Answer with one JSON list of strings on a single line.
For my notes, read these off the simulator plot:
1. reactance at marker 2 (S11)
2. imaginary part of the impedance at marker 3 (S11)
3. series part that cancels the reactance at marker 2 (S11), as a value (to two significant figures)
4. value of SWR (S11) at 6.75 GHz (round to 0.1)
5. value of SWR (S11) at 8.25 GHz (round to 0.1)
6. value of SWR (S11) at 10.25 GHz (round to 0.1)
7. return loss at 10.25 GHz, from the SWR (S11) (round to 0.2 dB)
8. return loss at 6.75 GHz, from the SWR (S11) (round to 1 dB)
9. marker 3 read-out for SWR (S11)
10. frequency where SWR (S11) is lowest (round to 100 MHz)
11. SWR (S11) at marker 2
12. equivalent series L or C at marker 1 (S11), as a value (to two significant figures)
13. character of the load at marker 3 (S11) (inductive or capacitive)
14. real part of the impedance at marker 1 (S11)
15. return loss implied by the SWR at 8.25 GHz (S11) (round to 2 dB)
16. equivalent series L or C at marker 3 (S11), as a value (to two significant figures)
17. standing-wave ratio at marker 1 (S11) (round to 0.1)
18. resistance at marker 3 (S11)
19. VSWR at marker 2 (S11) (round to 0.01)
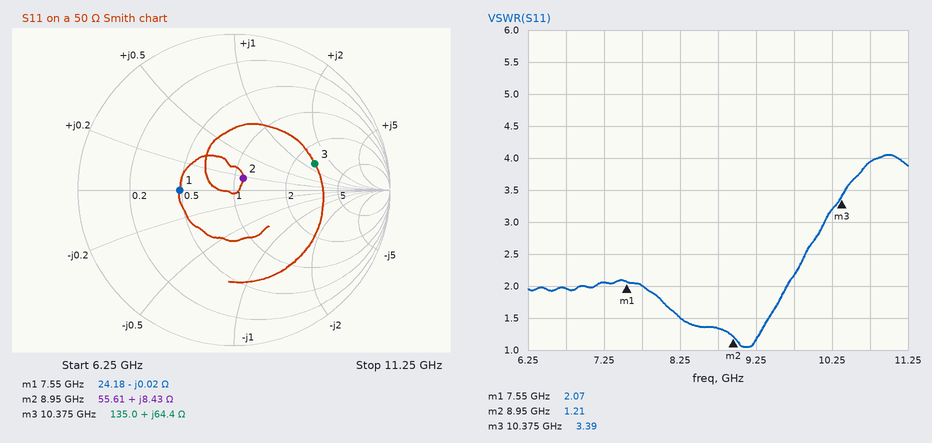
["+8.43 Ω", "+64.4 Ω", "2.1 pF", "2.0", "1.5", "3.2", "5.6 dB", "10 dB", "3.39", "9.1 GHz", "1.21", "1.1 nF", "inductive", "24.18 Ω", "14 dB", "990 pH", "2.1", "135.0 Ω", "1.21"]
